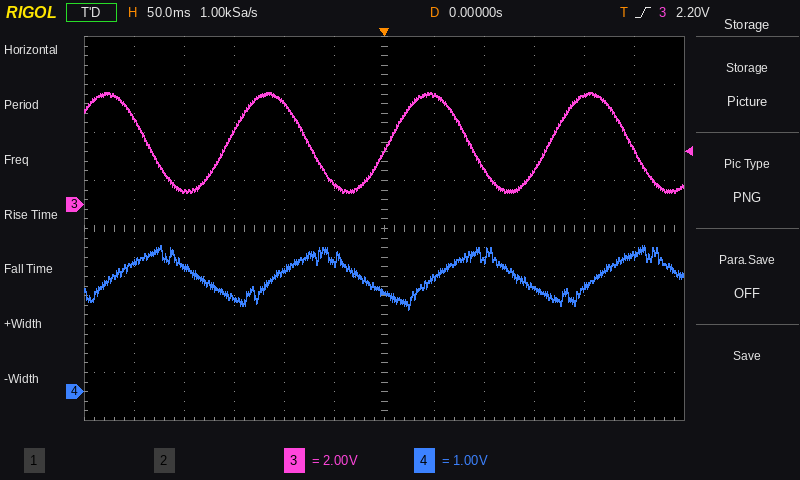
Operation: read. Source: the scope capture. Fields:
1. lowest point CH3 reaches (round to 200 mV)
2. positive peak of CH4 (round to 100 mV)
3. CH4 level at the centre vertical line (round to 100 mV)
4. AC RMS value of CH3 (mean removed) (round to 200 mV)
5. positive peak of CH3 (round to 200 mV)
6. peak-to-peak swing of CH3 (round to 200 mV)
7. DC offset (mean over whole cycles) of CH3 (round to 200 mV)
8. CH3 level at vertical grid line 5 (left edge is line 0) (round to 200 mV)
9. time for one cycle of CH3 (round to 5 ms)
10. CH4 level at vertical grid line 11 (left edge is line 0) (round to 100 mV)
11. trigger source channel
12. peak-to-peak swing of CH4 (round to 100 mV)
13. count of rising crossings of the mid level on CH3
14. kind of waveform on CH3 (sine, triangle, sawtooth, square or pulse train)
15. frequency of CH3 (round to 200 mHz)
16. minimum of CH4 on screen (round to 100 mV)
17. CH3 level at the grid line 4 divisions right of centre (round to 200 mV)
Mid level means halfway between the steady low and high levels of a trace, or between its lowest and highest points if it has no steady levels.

400 mV
3.0 V
2.1 V
1.4 V
4.6 V
4.2 V
2.6 V
800 mV
160 ms
2.8 V
CH3
1.3 V
3
sine
6.2 Hz
1.7 V
4.6 V
